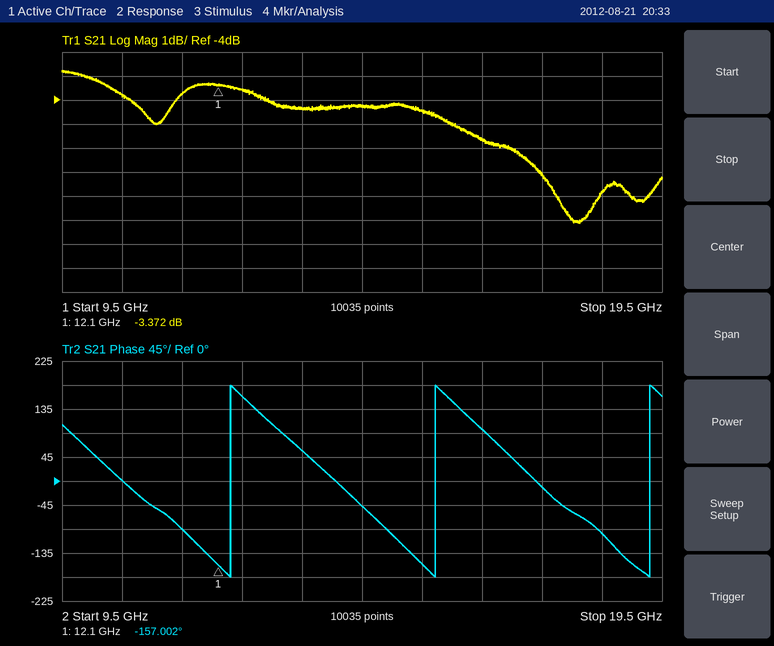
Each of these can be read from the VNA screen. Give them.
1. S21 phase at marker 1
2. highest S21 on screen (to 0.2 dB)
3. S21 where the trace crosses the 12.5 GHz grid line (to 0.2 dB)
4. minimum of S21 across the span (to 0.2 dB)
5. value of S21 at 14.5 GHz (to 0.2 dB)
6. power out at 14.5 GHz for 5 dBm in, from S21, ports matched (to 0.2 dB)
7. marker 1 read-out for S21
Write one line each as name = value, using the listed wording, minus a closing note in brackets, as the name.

S21 phase at marker 1 = -157.002°
highest S21 on screen = -2.8 dB
S21 where the trace crosses the 12.5 GHz grid line = -3.6 dB
minimum of S21 across the span = -9.2 dB
value of S21 at 14.5 GHz = -4.2 dB
power out at 14.5 GHz for 5 dBm in, from S21, ports matched = 0.8 dBm
marker 1 read-out for S21 = -3.372 dB
